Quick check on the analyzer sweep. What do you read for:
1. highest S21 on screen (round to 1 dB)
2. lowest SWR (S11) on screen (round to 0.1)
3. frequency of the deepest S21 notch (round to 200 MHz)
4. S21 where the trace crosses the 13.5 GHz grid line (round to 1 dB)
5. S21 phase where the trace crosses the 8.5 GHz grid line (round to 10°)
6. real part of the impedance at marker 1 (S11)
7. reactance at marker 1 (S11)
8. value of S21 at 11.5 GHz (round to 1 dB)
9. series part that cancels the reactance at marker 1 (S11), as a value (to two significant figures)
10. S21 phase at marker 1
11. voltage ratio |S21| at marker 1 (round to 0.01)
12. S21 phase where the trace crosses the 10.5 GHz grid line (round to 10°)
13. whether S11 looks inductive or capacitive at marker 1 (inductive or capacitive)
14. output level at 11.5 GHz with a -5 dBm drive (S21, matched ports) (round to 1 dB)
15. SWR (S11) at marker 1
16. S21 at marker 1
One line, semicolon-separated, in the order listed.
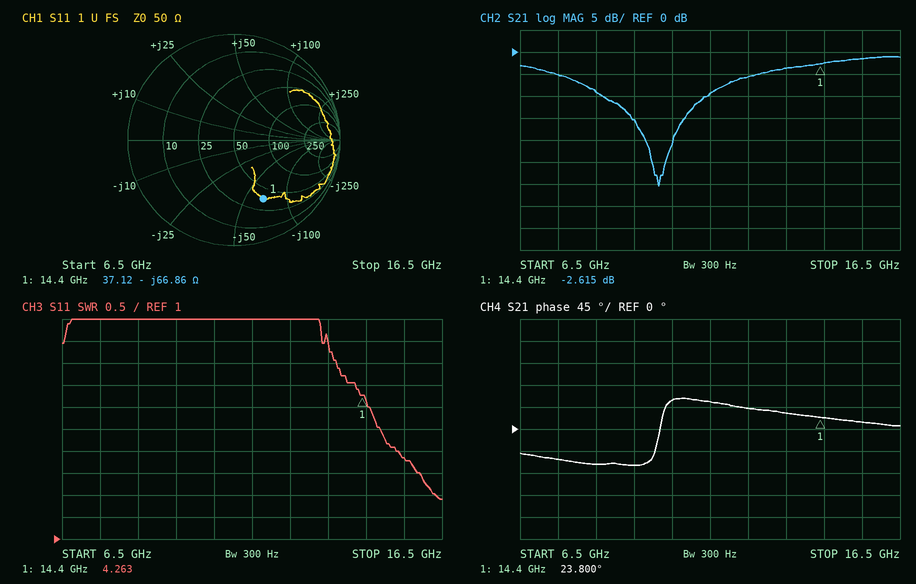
-1 dB; 1.9; 10.2 GHz; -4 dB; -70°; 37.12 Ω; -66.86 Ω; -9 dB; 740 pH; 23.800°; 0.74; 60°; capacitive; -14 dBm; 4.263; -2.615 dB
